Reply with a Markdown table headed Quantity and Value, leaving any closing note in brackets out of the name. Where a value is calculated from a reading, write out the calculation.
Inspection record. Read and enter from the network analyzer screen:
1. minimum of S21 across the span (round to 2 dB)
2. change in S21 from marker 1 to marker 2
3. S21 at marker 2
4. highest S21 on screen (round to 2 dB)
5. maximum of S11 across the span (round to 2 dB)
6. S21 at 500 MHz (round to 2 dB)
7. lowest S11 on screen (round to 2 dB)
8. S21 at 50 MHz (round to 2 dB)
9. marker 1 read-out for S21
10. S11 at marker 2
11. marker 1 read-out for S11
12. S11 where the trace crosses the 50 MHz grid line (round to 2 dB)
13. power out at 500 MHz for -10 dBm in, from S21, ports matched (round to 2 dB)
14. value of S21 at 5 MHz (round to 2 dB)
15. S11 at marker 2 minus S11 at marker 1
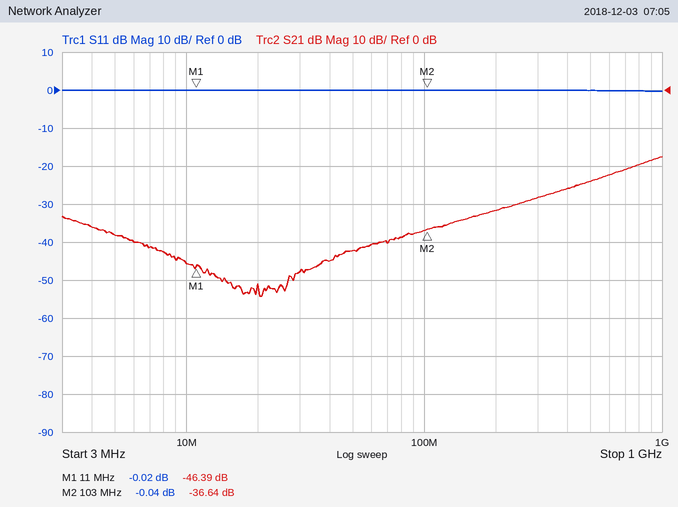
| Quantity | Value |
|---|---|
| minimum of S21 across the span | -54 dB |
| change in S21 from marker 1 to marker 2 | -36.64 − (-46.39) = 9.75 dB |
| S21 at marker 2 | -36.64 dB |
| highest S21 on screen | -18 dB |
| maximum of S11 across the span | 0 dB |
| S21 at 500 MHz | -24 dB |
| lowest S11 on screen | 0 dB |
| S21 at 50 MHz | -42 dB |
| marker 1 read-out for S21 | -46.39 dB |
| S11 at marker 2 | -0.04 dB |
| marker 1 read-out for S11 | -0.02 dB |
| S11 where the trace crosses the 50 MHz grid line | 0 dB |
| power out at 500 MHz for -10 dBm in, from S21, ports matched | -10 dBm + (-24 dB) = -34 dBm |
| value of S21 at 5 MHz | -38 dB |
| S11 at marker 2 minus S11 at marker 1 | -0.04 − (-0.02) = -0.02 dB |
